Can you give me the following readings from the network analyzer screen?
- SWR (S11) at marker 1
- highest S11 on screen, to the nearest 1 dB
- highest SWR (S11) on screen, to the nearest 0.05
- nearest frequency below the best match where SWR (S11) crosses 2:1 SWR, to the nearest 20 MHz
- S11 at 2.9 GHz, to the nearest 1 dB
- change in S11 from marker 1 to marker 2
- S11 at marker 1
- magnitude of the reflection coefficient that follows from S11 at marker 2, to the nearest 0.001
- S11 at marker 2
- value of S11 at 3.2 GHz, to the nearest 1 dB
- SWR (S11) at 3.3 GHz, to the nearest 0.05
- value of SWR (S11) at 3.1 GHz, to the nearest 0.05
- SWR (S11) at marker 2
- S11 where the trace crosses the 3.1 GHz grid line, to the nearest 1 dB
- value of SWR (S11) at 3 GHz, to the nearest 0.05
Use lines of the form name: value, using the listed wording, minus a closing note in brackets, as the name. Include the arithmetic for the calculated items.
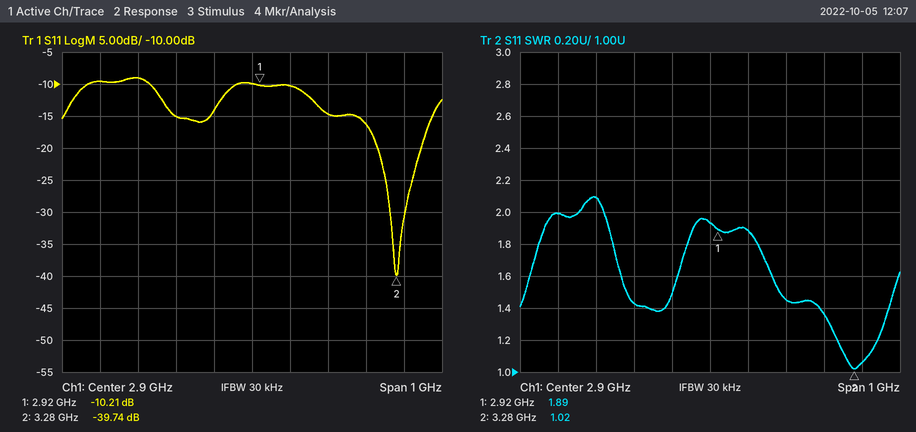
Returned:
SWR (S11) at marker 1: 1.89
highest S11 on screen, to the nearest 1 dB: -9 dB
highest SWR (S11) on screen, to the nearest 0.05: 2.10
nearest frequency below the best match where SWR (S11) crosses 2:1 SWR, to the nearest 20 MHz: 2.62 GHz
S11 at 2.9 GHz, to the nearest 1 dB: -10 dB
change in S11 from marker 1 to marker 2: -39.74 − (-10.21) = -29.53 dB
S11 at marker 1: -10.21 dB
magnitude of the reflection coefficient that follows from S11 at marker 2, to the nearest 0.001: 10^(-39.74/20) ≈ 0.010
S11 at marker 2: -39.74 dB
value of S11 at 3.2 GHz, to the nearest 1 dB: -16 dB
SWR (S11) at 3.3 GHz, to the nearest 0.05: 1.05
value of SWR (S11) at 3.1 GHz, to the nearest 0.05: 1.45
SWR (S11) at marker 2: 1.02
S11 where the trace crosses the 3.1 GHz grid line, to the nearest 1 dB: -15 dB
value of SWR (S11) at 3 GHz, to the nearest 0.05: 1.90
